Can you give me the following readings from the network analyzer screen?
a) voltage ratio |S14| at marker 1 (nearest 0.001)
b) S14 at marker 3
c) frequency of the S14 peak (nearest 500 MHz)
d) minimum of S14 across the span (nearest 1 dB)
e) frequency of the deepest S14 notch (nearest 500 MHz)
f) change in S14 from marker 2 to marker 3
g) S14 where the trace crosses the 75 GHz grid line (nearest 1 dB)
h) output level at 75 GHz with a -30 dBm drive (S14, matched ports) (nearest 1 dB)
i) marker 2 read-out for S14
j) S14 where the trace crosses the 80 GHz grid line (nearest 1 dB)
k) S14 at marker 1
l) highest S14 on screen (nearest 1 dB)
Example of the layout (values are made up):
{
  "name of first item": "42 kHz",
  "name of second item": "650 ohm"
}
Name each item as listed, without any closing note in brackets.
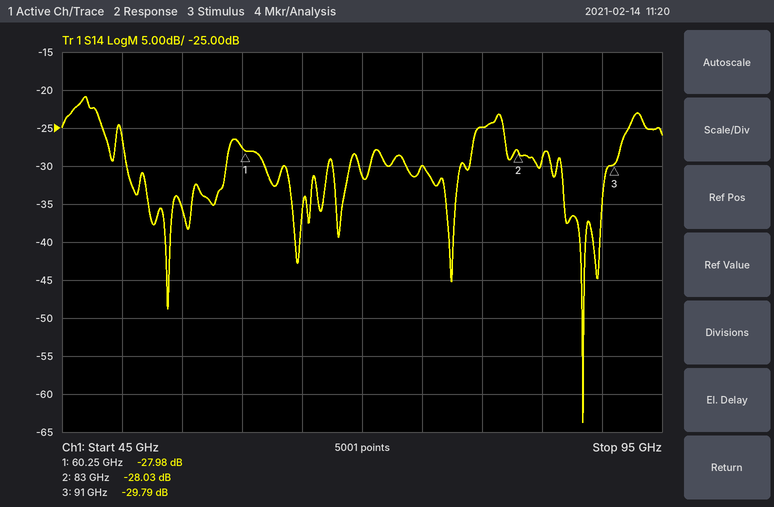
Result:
{
  "voltage ratio |S14| at marker 1": "0.040",
  "S14 at marker 3": "-29.79 dB",
  "frequency of the S14 peak": "47.0 GHz",
  "minimum of S14 across the span": "-64 dB",
  "frequency of the deepest S14 notch": "88.5 GHz",
  "change in S14 from marker 2 to marker 3": "-1.76 dB",
  "S14 where the trace crosses the 75 GHz grid line": "-30 dB",
  "output level at 75 GHz with a -30 dBm drive (S14, matched ports)": "-60 dBm",
  "marker 2 read-out for S14": "-28.03 dB",
  "S14 where the trace crosses the 80 GHz grid line": "-25 dB",
  "S14 at marker 1": "-27.98 dB",
  "highest S14 on screen": "-21 dB"
}
